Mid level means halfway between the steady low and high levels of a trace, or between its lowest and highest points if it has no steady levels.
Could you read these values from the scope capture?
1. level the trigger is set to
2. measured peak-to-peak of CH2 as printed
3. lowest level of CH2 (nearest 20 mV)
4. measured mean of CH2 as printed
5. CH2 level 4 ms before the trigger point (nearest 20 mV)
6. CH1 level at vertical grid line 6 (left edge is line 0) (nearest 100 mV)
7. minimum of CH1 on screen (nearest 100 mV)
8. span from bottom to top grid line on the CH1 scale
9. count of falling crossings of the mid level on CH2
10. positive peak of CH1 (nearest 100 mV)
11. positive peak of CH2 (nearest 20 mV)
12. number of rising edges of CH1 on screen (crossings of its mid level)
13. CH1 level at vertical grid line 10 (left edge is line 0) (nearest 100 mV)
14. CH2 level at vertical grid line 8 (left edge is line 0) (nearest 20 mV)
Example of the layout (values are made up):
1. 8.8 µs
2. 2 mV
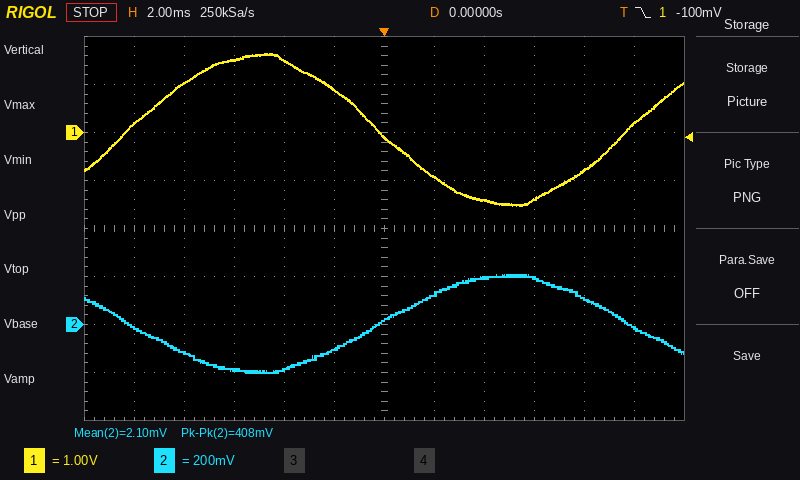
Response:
1. -100 mV
2. 408 mV
3. -200 mV
4. 2.10 mV
5. -180 mV
6. -100 mV
7. -1.5 V
8. 8 V
9. 2
10. 1.6 V
11. 200 mV
12. 2
13. -800 mV
14. 200 mV
